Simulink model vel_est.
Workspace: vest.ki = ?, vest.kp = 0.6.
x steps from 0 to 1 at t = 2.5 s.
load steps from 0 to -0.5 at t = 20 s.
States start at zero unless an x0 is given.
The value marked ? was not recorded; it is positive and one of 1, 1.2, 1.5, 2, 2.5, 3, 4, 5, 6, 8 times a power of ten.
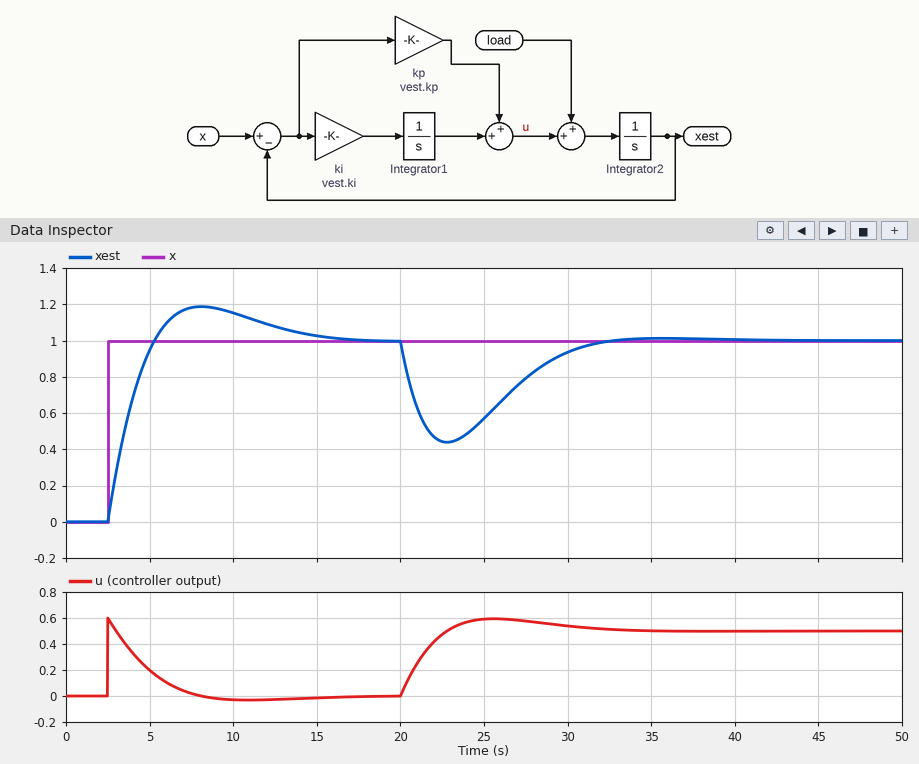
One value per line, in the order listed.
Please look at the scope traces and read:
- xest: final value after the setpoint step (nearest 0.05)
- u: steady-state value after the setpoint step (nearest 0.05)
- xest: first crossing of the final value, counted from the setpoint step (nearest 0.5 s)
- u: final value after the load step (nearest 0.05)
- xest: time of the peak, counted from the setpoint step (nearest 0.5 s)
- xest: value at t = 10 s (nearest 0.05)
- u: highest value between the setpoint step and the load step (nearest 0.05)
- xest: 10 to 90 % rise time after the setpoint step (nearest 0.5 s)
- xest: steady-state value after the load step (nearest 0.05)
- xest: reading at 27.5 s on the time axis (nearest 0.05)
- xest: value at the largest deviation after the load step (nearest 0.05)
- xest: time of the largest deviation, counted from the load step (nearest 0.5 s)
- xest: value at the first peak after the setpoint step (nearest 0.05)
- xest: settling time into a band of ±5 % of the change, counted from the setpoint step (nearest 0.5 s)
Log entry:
1.00
0.00
3.0 s
0.50
5.5 s
1.15
0.60
2.0 s
1.00
0.80
0.45
3.0 s
1.20
11.0 s
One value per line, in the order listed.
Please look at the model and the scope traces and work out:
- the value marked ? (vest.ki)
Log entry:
0.15
